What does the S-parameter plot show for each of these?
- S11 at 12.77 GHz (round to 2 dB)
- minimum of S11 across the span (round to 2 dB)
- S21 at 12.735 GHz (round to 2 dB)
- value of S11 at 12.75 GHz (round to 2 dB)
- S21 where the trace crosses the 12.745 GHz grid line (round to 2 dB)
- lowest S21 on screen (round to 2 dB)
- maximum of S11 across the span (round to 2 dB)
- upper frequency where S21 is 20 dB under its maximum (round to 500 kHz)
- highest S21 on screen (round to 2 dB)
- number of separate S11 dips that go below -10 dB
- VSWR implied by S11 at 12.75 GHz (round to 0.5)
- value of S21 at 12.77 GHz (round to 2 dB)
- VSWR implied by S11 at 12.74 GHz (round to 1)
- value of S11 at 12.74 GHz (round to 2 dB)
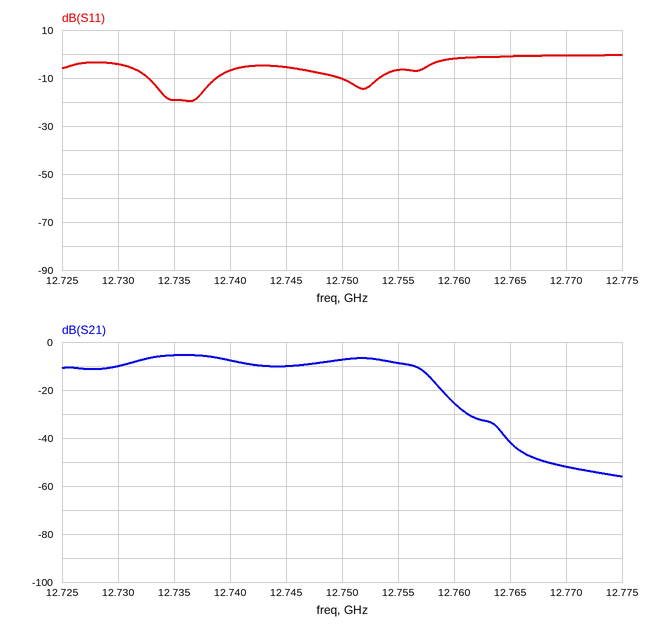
0 dB
-20 dB
-6 dB
-10 dB
-10 dB
-56 dB
0 dB
12.7600 GHz
-6 dB
2
2.0
-52 dB
3
-6 dB
